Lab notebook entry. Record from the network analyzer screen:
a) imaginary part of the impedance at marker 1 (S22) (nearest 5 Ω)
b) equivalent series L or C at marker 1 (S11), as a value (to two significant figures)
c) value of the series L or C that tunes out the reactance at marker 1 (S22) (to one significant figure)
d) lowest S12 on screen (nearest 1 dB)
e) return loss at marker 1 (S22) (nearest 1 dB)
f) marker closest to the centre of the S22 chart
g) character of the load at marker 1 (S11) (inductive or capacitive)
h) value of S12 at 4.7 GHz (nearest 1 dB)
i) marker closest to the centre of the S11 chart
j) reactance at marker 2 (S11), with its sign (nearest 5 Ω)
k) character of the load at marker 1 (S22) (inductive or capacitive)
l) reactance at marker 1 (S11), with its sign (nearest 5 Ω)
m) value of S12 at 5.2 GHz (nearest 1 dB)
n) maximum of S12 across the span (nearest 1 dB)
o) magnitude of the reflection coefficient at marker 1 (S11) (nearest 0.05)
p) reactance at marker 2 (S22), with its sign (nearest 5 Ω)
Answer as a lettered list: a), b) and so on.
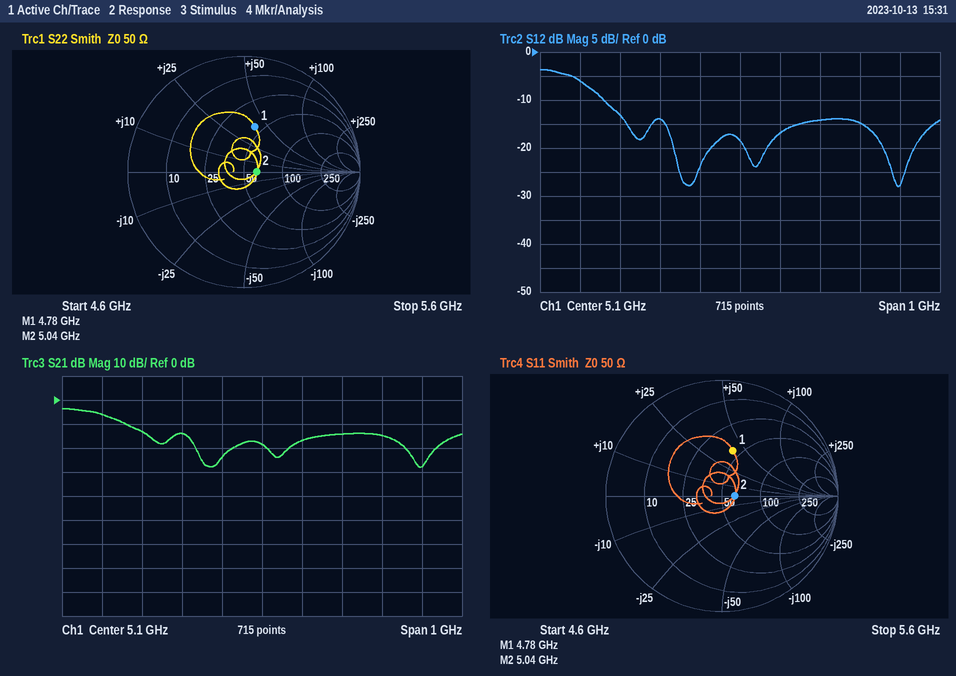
a) +40 Ω
b) 1.3 nH
c) 800 fF
d) -28 dB
e) 8 dB
f) marker 2
g) inductive
h) -6 dB
i) marker 2
j) 0 Ω
k) inductive
l) +40 Ω
m) -17 dB
n) -4 dB
o) 0.40
p) 0 Ω
